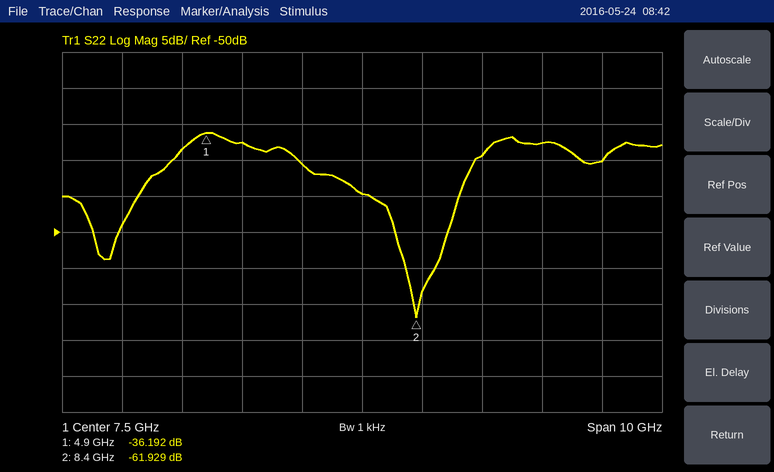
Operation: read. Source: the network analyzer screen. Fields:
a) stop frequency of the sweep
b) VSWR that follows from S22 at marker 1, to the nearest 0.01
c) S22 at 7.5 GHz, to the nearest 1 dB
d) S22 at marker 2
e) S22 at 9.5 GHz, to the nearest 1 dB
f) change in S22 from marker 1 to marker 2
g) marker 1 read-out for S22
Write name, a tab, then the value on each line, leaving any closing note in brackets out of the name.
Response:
stop frequency of the sweep	12.5 GHz
VSWR that follows from S22 at marker 1, to the nearest 0.01	1.03
S22 at 7.5 GHz, to the nearest 1 dB	-45 dB
S22 at marker 2	-61.929 dB
S22 at 9.5 GHz, to the nearest 1 dB	-39 dB
change in S22 from marker 1 to marker 2	-25.737 dB
marker 1 read-out for S22	-36.192 dB
